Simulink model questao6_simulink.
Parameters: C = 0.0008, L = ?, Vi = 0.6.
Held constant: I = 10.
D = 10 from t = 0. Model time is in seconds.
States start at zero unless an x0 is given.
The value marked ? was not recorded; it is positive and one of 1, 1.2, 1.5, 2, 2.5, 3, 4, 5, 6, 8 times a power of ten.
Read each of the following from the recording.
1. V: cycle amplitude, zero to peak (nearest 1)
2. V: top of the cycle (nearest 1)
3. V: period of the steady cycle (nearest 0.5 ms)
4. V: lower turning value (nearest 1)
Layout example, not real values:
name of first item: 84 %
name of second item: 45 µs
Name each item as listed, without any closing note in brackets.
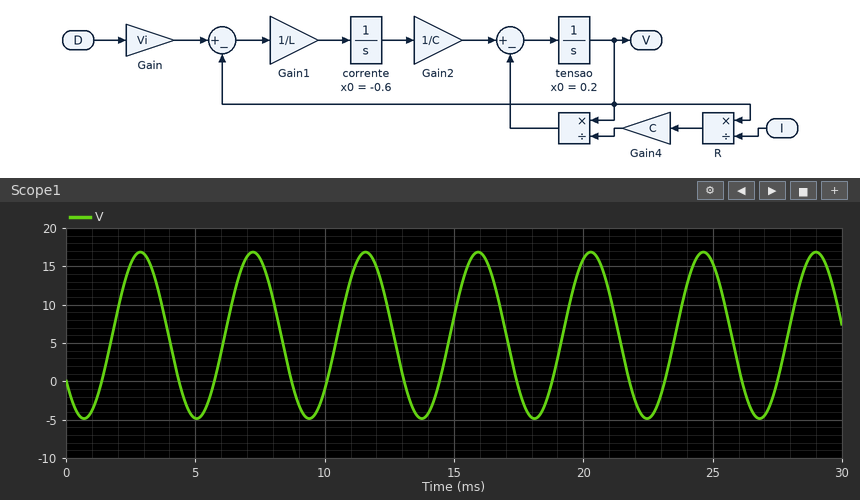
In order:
V: cycle amplitude, zero to peak: 11
V: top of the cycle: 17
V: period of the steady cycle: 4.5 ms
V: lower turning value: -5
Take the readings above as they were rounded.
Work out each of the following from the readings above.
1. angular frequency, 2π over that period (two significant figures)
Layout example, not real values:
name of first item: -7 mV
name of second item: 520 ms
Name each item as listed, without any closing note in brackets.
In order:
angular frequency, 2π over that period: 1.4 rad/ms
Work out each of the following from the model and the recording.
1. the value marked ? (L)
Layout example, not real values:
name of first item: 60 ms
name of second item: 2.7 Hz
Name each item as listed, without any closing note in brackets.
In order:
the value marked ?: 0.0006
